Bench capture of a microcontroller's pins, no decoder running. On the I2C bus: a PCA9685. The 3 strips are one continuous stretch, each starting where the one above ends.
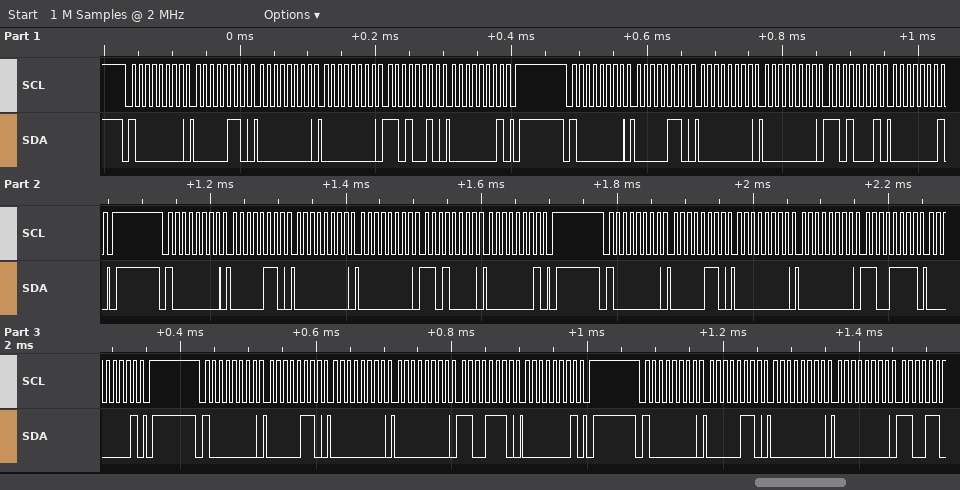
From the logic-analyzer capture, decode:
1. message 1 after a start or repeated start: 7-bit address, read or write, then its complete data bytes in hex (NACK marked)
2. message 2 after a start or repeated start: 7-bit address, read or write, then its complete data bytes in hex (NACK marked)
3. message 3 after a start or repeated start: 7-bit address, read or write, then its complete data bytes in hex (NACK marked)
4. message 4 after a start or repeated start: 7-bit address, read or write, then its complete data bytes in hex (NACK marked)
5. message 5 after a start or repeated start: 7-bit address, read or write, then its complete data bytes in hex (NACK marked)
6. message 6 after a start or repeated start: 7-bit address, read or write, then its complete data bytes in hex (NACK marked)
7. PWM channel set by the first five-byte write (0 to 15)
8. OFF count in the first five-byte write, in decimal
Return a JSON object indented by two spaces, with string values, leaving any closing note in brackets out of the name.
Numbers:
{
  "message 1 after a start or repeated start: 7-bit address, read or write, then its complete data bytes in hex": "0x40 write: 06 00 00 D2 01",
  "message 2 after a start or repeated start: 7-bit address, read or write, then its complete data bytes in hex": "0x40 write: 06 00 00 D1 01",
  "message 3 after a start or repeated start: 7-bit address, read or write, then its complete data bytes in hex": "0x40 write: 06 00 00 D0 01",
  "message 4 after a start or repeated start: 7-bit address, read or write, then its complete data bytes in hex": "0x40 write: 06 00 00 CF 01",
  "message 5 after a start or repeated start: 7-bit address, read or write, then its complete data bytes in hex": "0x40 write: 06 00 00 CE 01",
  "message 6 after a start or repeated start: 7-bit address, read or write, then its complete data bytes in hex": "0x40 write: 06 00 00",
  "PWM channel set by the first five-byte write": "0",
  "OFF count in the first five-byte write, in decimal": "466"
}
